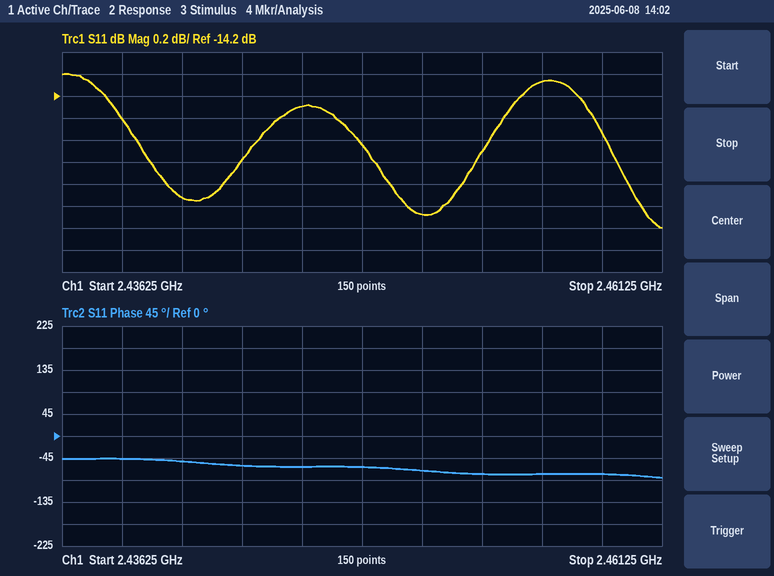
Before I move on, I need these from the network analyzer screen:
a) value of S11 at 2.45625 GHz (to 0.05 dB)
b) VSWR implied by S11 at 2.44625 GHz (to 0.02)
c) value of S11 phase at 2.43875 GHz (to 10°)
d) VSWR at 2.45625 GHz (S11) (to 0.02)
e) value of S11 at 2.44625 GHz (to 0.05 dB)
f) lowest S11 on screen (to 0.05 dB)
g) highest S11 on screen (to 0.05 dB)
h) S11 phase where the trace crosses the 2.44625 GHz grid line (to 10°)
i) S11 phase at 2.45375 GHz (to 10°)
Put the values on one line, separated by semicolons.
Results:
-14.05 dB; 1.48; -50°; 1.50; -14.30 dB; -15.40 dB; -14.00 dB; -60°; -80°
